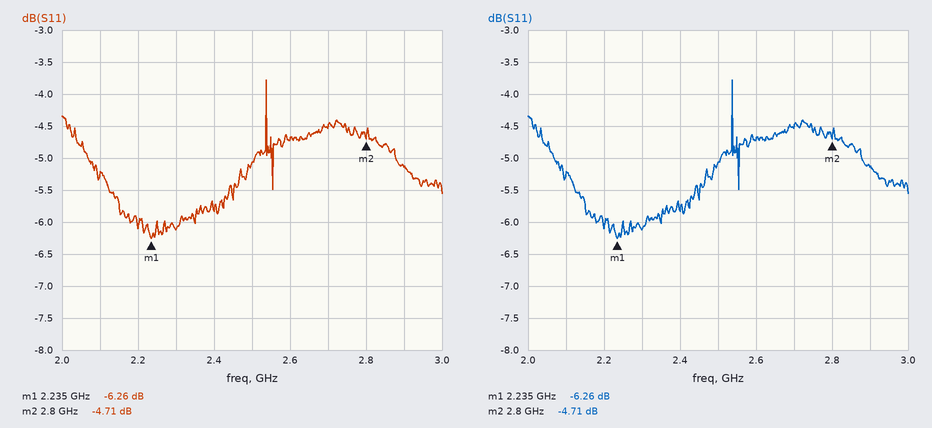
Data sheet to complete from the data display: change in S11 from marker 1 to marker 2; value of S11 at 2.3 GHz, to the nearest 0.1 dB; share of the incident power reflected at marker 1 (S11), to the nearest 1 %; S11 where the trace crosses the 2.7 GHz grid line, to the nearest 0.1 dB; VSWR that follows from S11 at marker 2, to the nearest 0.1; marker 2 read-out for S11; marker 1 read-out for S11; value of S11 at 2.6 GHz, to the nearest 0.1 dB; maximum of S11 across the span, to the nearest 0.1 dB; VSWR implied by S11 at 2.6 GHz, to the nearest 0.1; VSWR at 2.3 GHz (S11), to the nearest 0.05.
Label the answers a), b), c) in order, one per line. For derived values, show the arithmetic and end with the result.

a) -4.71 − (-6.26) = 1.55 dB
b) -6.1 dB
c) 10^(-6.26/10) ≈ 24 %
d) -4.5 dB
e) (1 + 0.5814)/(1 − 0.5814) ≈ 3.8
f) -4.71 dB
g) -6.26 dB
h) -4.7 dB
i) -3.8 dB
j) |Γ| = 10^(-4.7/20) = 0.5821; VSWR = (1 + 0.5821)/(1 − 0.5821) ≈ 3.8
k) |Γ| = 10^(-6.1/20) = 0.4955; VSWR = (1 + 0.4955)/(1 − 0.4955) ≈ 2.96, so 2.95 to the nearest 0.05
